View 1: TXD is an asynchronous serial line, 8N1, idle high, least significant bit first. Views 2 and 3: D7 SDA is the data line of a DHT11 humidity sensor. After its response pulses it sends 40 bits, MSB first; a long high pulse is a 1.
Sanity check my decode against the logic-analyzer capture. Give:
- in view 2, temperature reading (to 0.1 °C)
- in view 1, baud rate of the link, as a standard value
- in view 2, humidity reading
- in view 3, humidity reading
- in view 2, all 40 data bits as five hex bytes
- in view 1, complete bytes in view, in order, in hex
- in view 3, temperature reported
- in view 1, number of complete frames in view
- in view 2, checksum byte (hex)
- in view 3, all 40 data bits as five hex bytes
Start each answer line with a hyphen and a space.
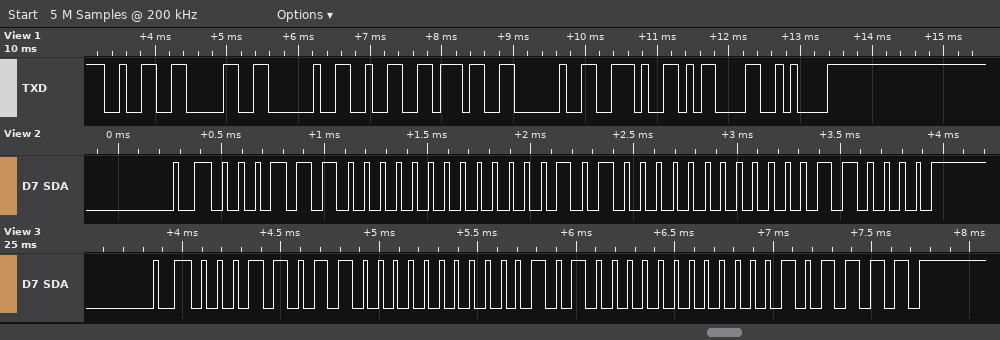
- 20.0 °C
- 9600 baud
- 28 %
- 27 %
- 1C 00 14 00 30
- 32 30 20 32 37 20 2E 0D 0A
- 20.0 °C
- 9
- 0x30
- 1B 00 14 00 2F
